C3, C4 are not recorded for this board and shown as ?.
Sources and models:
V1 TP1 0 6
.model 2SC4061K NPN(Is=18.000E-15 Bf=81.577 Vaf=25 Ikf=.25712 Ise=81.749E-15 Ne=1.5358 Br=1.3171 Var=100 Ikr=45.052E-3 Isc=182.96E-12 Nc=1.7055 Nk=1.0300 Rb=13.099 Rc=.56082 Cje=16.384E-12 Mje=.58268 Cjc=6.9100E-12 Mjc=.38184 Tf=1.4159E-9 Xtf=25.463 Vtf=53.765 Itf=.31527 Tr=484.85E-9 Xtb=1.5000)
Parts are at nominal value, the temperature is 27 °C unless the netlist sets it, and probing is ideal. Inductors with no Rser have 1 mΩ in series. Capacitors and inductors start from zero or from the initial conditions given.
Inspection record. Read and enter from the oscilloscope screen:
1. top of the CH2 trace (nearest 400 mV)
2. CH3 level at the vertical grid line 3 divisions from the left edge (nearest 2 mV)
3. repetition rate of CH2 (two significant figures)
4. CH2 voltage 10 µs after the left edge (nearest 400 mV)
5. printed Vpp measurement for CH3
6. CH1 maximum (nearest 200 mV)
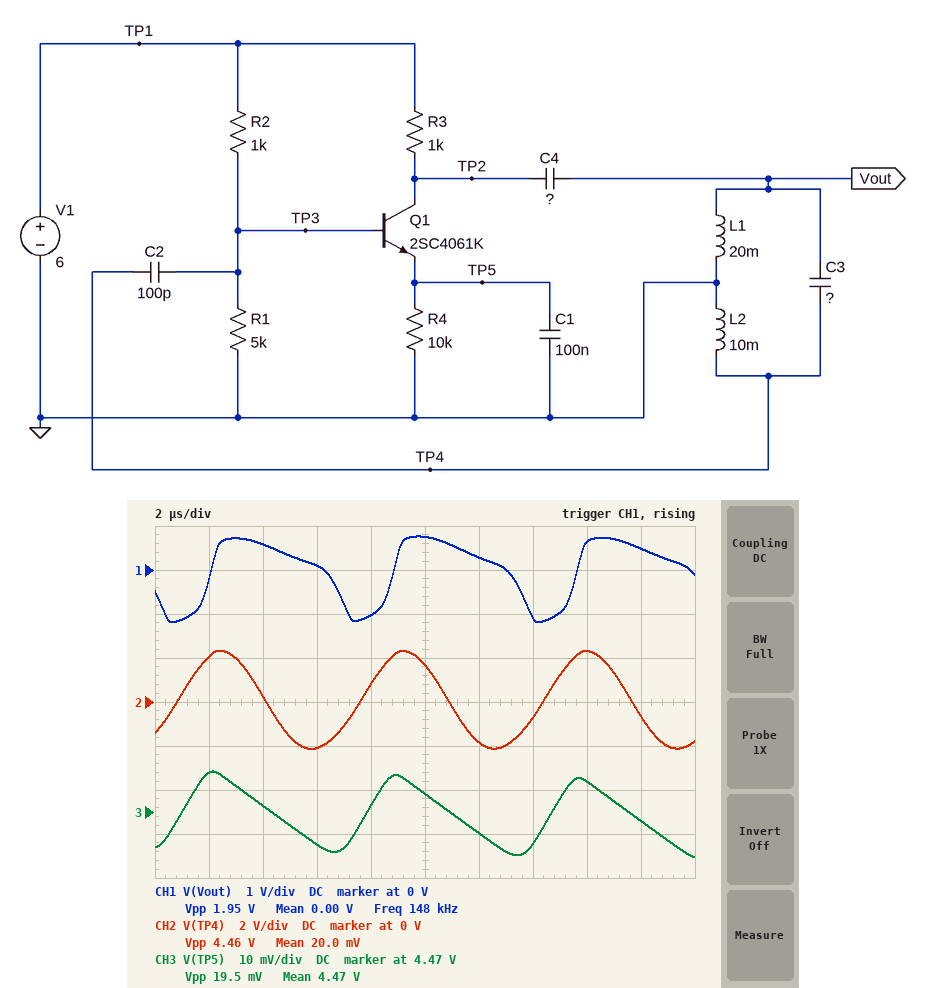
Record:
2.4 V
4.462 V
150 kHz
1.6 V
19.5 mV
800 mV
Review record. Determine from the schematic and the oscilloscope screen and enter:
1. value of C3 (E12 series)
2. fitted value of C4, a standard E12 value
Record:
18 pF
180 pF
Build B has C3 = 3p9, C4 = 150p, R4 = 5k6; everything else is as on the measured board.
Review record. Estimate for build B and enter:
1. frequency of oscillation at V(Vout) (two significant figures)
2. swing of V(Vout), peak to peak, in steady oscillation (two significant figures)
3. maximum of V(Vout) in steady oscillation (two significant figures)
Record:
160 kHz
2.3 V
1.1 V
